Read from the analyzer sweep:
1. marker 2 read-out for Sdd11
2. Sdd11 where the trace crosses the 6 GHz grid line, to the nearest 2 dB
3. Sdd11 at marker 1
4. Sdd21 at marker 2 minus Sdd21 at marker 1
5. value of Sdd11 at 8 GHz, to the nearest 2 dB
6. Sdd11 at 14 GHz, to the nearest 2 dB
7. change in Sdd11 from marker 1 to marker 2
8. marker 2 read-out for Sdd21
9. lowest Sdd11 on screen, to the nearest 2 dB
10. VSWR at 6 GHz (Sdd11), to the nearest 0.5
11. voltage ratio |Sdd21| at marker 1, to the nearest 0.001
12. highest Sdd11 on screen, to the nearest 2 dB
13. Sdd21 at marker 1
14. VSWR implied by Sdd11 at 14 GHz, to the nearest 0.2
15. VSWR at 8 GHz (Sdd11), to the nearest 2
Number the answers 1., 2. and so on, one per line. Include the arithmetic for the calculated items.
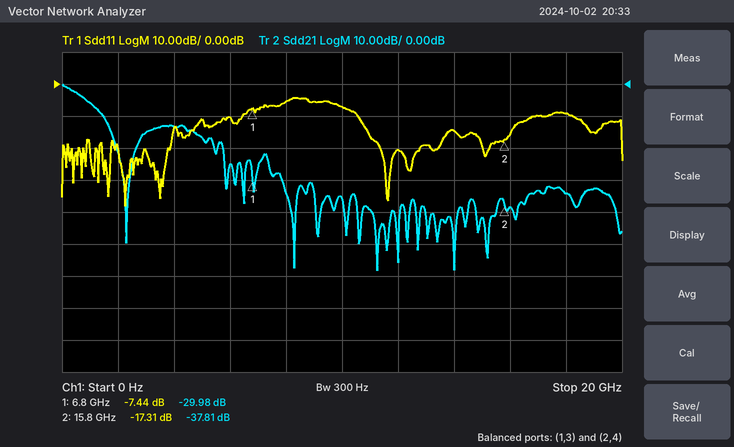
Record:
1. -17.31 dB
2. -10 dB
3. -7.44 dB
4. -37.81 − (-29.98) = -7.83 dB
5. -6 dB
6. -14 dB
7. -17.31 − (-7.44) = -9.87 dB
8. -37.81 dB
9. -38 dB
10. |Γ| = 10^(-10/20) = 0.3162; VSWR = (1 + 0.3162)/(1 − 0.3162) ≈ 1.92, so 2.0 to the nearest 0.5
11. 10^(-29.98/20) ≈ 0.032
12. -4 dB
13. -29.98 dB
14. |Γ| = 10^(-14/20) = 0.1995; VSWR = (1 + 0.1995)/(1 − 0.1995) ≈ 1.50, so 1.4 to the nearest 0.2
15. |Γ| = 10^(-6/20) = 0.5012; VSWR = (1 + 0.5012)/(1 − 0.5012) ≈ 3.01, so 4 to the nearest 2
